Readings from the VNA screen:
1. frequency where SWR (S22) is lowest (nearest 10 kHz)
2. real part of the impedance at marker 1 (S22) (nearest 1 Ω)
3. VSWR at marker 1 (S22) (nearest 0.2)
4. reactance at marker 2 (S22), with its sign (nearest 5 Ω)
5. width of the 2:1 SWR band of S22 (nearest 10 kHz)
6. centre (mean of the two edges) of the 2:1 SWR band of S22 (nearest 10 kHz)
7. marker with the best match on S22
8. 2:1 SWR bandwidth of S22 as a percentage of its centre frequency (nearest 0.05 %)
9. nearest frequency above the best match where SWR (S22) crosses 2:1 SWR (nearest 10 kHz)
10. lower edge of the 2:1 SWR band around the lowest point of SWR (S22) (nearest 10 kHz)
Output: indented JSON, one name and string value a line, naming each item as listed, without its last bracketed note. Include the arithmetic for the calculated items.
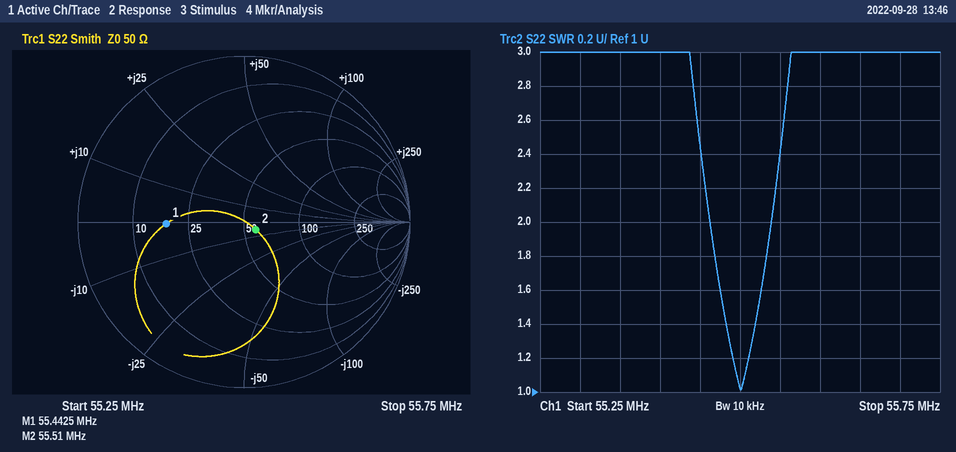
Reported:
{
  "frequency where SWR (S22) is lowest": "55.50 MHz",
  "real part of the impedance at marker 1 (S22)": "18 Ω",
  "VSWR at marker 1 (S22)": "2.8",
  "reactance at marker 2 (S22), with its sign": "-5 Ω",
  "width of the 2:1 SWR band of S22": "55.54 MHz − 55.46 MHz = 80 kHz",
  "centre (mean of the two edges) of the 2:1 SWR band of S22": "55.50 MHz",
  "marker with the best match on S22": "marker 2",
  "2:1 SWR bandwidth of S22 as a percentage of its centre frequency": "80 kHz / 55.5 MHz ≈ 0.144 %, so 0.15 % to the nearest 0.05 %",
  "nearest frequency above the best match where SWR (S22) crosses 2:1 SWR": "55.54 MHz",
  "lower edge of the 2:1 SWR band around the lowest point of SWR (S22)": "55.46 MHz"
}
